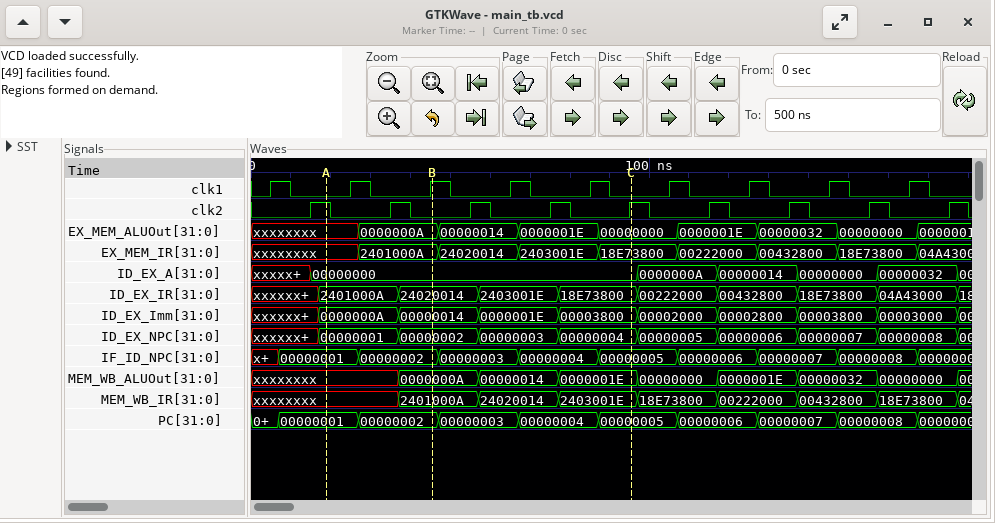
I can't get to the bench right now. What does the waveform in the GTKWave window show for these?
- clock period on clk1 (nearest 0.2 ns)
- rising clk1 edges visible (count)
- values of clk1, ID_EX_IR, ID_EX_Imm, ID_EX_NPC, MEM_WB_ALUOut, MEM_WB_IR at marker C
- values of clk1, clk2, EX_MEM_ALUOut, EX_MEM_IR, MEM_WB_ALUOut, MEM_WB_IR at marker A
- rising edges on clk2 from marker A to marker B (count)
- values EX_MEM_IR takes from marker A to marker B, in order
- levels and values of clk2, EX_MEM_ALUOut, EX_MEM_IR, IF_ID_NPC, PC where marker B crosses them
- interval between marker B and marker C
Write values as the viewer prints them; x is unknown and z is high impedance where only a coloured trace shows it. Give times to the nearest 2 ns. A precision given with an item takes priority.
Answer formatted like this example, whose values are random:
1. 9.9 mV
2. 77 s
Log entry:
1. 20 ns
2. 9
3. clk1=0, ID_EX_IR=18E73800, ID_EX_Imm=00003800, ID_EX_NPC=00000004, MEM_WB_ALUOut=0000001E, MEM_WB_IR=2403001E
4. clk1=0, clk2=1, EX_MEM_ALUOut=xxxxxxxx, EX_MEM_IR=xxxxxxxx, MEM_WB_ALUOut=xxxxxxxx, MEM_WB_IR=xxxxxxxx
5. 1
6. xxxxxxxx, 2401000A
7. clk2=0, EX_MEM_ALUOut=0000000A, EX_MEM_IR=2401000A, IF_ID_NPC=00000002, PC=00000002
8. 50 ns
